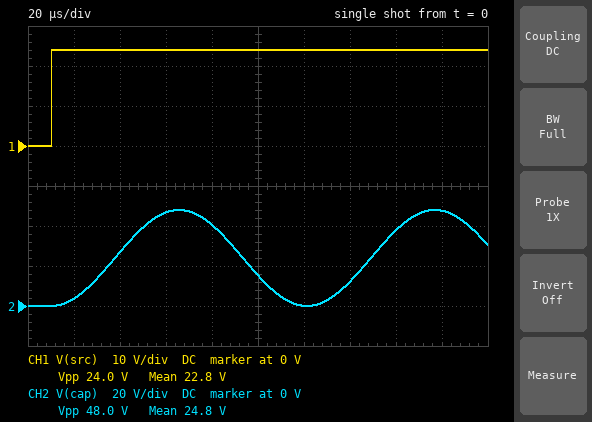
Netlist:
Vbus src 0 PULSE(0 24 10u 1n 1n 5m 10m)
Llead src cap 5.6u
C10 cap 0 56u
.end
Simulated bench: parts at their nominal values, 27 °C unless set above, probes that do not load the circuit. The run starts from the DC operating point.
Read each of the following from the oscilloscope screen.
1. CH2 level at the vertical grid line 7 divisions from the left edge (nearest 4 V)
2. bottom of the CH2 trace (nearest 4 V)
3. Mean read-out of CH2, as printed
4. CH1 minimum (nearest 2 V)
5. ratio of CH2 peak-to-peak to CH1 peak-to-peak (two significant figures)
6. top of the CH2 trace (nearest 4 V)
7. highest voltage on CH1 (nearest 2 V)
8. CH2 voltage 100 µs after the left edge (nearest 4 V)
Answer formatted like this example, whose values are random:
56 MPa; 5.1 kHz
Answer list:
12 V; 0 V; 24.8 V; 0 V; 2.0; 48 V; 24 V; 16 V
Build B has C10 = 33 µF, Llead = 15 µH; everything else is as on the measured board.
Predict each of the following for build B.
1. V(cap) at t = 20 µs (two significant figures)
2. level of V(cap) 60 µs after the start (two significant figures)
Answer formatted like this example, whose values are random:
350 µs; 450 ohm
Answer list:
2.4 V; 39 V
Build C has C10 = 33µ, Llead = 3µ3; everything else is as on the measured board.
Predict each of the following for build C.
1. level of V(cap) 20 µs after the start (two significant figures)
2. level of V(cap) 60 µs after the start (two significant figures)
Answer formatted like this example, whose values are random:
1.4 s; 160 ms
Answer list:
10 V; 22 V
